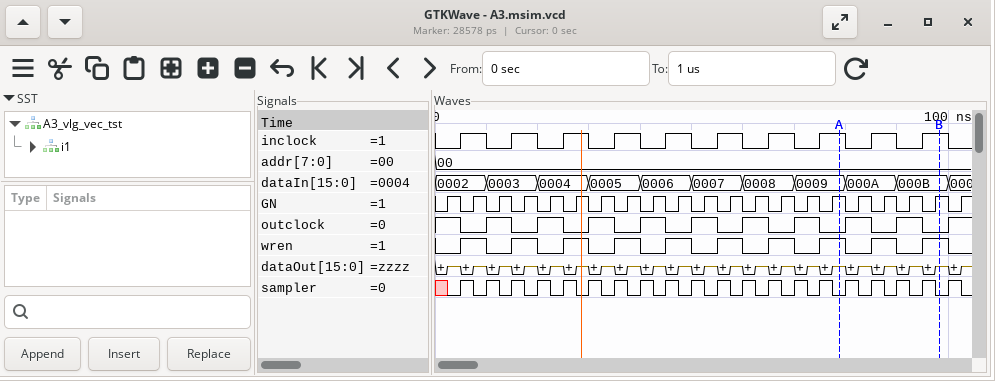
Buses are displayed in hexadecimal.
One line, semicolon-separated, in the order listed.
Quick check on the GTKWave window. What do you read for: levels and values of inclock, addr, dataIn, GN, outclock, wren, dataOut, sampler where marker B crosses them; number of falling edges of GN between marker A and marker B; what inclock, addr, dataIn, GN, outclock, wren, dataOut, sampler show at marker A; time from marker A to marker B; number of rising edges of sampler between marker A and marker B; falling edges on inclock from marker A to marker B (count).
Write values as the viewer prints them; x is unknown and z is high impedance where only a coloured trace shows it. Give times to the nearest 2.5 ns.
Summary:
inclock=1, addr=00, dataIn=000B, GN=1, outclock=0, wren=1, dataOut=z, sampler=0; 4; inclock=1, addr=00, dataIn=0009, GN=1, outclock=0, wren=1, dataOut=z, sampler=0; 20 ns; 4; 2
